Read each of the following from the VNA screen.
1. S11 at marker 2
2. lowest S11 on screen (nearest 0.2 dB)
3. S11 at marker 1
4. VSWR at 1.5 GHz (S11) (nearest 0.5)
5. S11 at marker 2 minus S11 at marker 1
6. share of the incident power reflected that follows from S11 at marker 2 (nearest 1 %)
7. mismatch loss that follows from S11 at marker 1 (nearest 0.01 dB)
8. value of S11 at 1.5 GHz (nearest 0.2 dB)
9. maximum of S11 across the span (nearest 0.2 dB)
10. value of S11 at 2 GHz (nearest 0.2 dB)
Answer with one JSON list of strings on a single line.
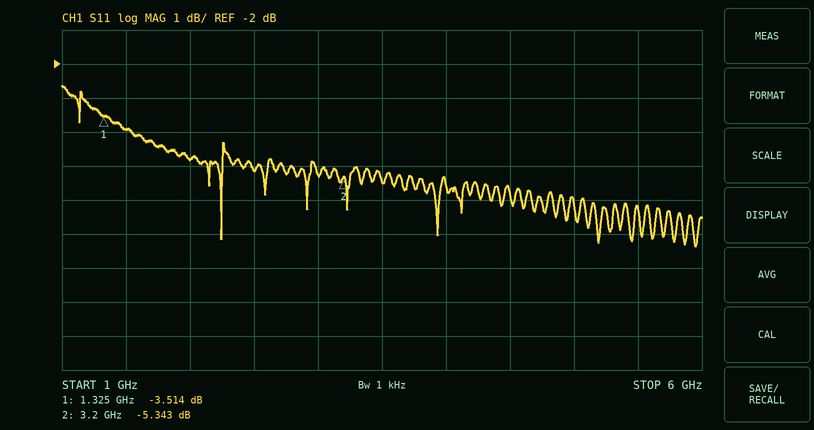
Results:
["-5.343 dB", "-7.4 dB", "-3.514 dB", "4.5", "-1.829 dB", "29 %", "2.56 dB", "-4.0 dB", "-2.6 dB", "-4.8 dB"]
